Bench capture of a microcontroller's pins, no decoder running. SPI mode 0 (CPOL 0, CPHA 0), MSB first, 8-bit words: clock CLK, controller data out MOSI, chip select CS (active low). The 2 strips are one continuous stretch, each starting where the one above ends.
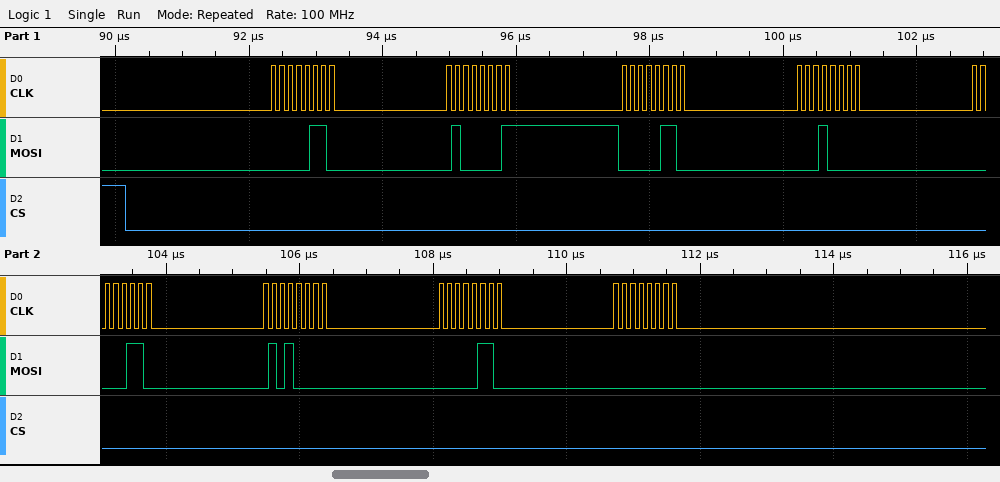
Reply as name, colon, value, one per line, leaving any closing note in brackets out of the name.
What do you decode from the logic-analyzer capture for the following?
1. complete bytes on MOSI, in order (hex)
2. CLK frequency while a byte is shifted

complete bytes on MOSI, in order: 0x06 0x41 0x06 0x10 0x06 0x50 0x06 0x00
CLK frequency while a byte is shifted: 8 MHz
